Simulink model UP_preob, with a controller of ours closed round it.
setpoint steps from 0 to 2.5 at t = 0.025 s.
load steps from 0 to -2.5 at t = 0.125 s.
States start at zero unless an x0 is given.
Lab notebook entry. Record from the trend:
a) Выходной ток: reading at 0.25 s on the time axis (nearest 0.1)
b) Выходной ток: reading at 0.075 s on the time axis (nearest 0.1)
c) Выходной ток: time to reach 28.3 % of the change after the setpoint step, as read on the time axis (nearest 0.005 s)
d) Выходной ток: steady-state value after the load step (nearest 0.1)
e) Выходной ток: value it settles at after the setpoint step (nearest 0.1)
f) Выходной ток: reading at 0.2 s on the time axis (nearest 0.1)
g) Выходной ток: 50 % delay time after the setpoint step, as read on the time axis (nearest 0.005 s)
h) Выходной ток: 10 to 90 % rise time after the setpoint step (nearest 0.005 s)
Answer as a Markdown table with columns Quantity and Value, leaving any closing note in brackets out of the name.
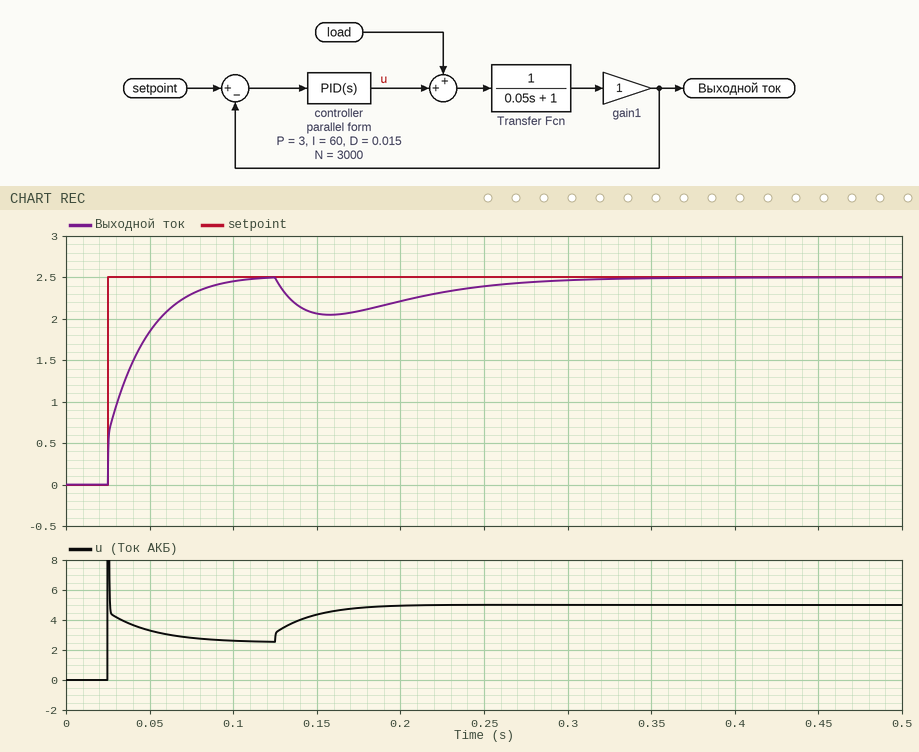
| Quantity | Value |
|---|---|
| Выходной ток: reading at 0.25 s on the time axis | 2.4 |
| Выходной ток: reading at 0.075 s on the time axis | 2.3 |
| Выходной ток: time to reach 28.3 % of the change after the setpoint step, as read on the time axis | 0.025 s |
| Выходной ток: steady-state value after the load step | 2.5 |
| Выходной ток: value it settles at after the setpoint step | 2.5 |
| Выходной ток: reading at 0.2 s on the time axis | 2.2 |
| Выходной ток: 50 % delay time after the setpoint step, as read on the time axis | 0.035 s |
| Выходной ток: 10 to 90 % rise time after the setpoint step | 0.045 s |
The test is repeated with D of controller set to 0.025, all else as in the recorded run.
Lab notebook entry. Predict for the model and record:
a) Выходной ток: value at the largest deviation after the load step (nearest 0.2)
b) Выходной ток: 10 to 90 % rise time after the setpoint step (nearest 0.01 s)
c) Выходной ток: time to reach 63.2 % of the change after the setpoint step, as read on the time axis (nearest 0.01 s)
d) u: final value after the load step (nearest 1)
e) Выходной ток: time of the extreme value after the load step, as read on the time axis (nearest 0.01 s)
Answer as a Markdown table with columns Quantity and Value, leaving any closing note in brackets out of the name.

| Quantity | Value |
|---|---|
| Выходной ток: value at the largest deviation after the load step | 2.0 |
| Выходной ток: 10 to 90 % rise time after the setpoint step | 0.05 s |
| Выходной ток: time to reach 63.2 % of the change after the setpoint step, as read on the time axis | 0.04 s |
| u: final value after the load step | 5 |
| Выходной ток: time of the extreme value after the load step, as read on the time axis | 0.16 s |
